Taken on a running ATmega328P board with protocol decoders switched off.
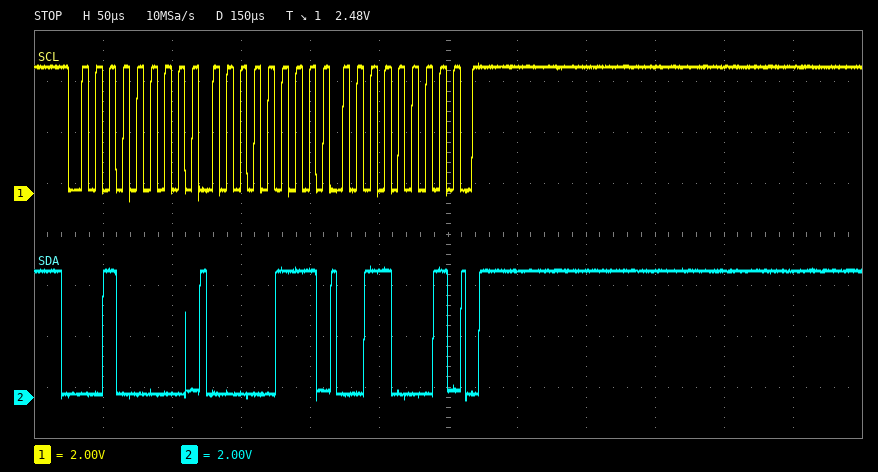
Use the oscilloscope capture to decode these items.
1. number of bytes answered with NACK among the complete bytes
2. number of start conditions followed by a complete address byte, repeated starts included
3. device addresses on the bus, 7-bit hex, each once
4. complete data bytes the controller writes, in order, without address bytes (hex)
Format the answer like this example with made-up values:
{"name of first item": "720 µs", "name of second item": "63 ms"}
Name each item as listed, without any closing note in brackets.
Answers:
{"number of bytes answered with NACK among the complete bytes": "0", "number of start conditions followed by a complete address byte, repeated starts included": "1", "device addresses on the bus, 7-bit hex, each once": "0x10", "complete data bytes the controller writes, in order, without address bytes": "07 31"}
